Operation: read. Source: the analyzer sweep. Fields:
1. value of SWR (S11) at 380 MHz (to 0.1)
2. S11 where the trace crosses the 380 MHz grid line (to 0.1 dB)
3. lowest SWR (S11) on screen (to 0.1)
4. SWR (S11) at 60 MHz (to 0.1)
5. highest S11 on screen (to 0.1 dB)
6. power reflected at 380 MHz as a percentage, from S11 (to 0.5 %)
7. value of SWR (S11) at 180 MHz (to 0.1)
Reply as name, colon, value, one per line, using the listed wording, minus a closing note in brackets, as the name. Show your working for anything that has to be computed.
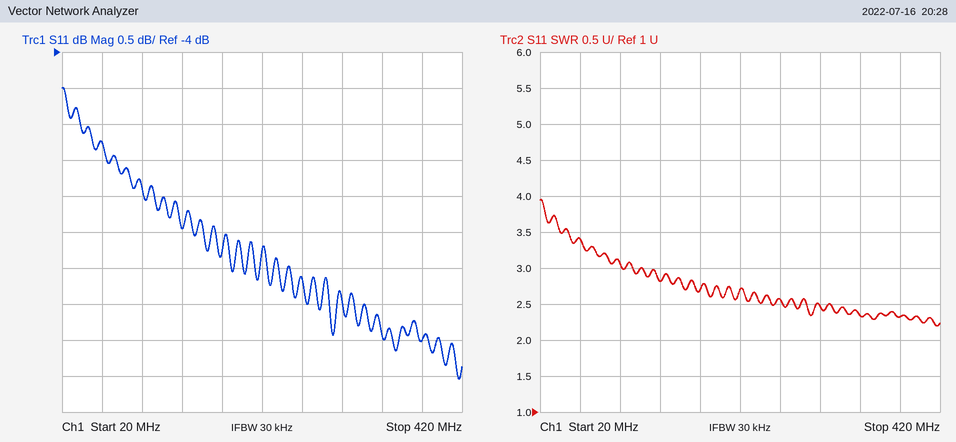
value of SWR (S11) at 380 MHz: 2.3
S11 where the trace crosses the 380 MHz grid line: -8.0 dB
lowest SWR (S11) on screen: 2.2
SWR (S11) at 60 MHz: 3.4
highest S11 on screen: -4.5 dB
power reflected at 380 MHz as a percentage, from S11: 10^(-8/10) ≈ 15.8 %, so 16.0 % to the nearest 0.5 %
value of SWR (S11) at 180 MHz: 2.7
